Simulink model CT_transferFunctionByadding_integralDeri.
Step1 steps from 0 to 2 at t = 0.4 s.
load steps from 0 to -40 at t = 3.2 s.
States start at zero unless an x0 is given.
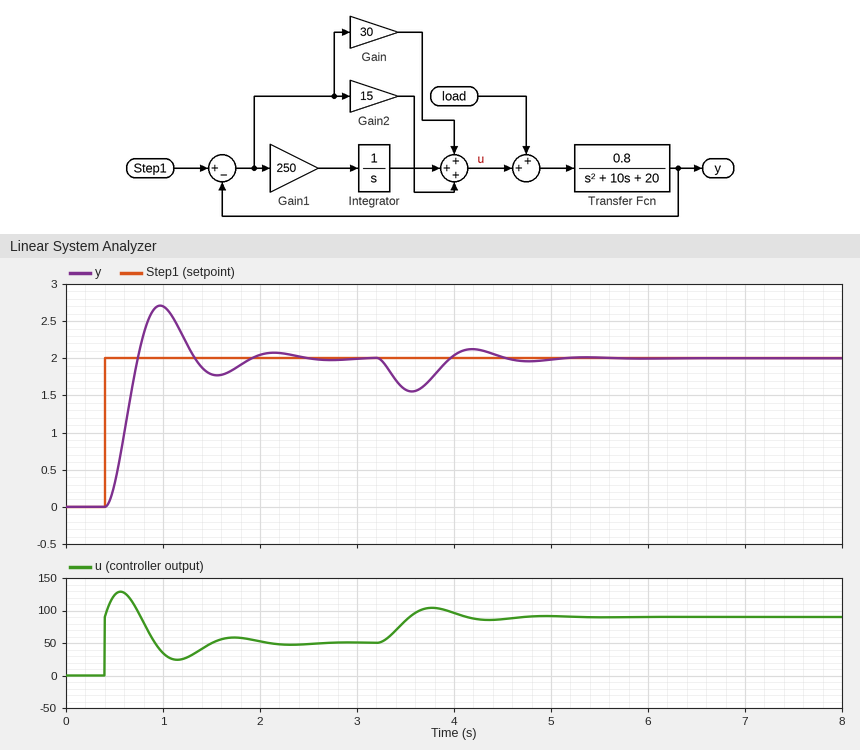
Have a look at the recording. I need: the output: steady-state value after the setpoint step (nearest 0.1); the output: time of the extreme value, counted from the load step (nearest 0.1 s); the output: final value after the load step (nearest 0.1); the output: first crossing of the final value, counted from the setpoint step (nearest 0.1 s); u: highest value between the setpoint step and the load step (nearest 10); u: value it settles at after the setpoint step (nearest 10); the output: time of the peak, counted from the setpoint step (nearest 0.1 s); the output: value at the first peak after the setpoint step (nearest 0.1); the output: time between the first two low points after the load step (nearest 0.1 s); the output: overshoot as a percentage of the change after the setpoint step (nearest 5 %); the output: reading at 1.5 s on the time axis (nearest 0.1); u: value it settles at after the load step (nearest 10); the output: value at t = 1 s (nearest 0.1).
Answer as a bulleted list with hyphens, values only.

- 2.0
- 0.4 s
- 2.0
- 0.3 s
- 130
- 50
- 0.6 s
- 2.7
- 1.2 s
- 35 %
- 1.8
- 90
- 2.7
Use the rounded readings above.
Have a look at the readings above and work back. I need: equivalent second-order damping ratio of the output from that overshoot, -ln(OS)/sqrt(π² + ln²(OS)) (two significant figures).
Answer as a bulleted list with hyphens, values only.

- 0.32
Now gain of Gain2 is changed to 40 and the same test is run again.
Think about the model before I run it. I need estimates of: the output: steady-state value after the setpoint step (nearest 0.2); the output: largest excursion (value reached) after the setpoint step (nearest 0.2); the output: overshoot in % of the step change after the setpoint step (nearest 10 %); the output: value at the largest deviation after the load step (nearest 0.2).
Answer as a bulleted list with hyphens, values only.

- 2.0
- 2.6
- 30 %
- 1.6
